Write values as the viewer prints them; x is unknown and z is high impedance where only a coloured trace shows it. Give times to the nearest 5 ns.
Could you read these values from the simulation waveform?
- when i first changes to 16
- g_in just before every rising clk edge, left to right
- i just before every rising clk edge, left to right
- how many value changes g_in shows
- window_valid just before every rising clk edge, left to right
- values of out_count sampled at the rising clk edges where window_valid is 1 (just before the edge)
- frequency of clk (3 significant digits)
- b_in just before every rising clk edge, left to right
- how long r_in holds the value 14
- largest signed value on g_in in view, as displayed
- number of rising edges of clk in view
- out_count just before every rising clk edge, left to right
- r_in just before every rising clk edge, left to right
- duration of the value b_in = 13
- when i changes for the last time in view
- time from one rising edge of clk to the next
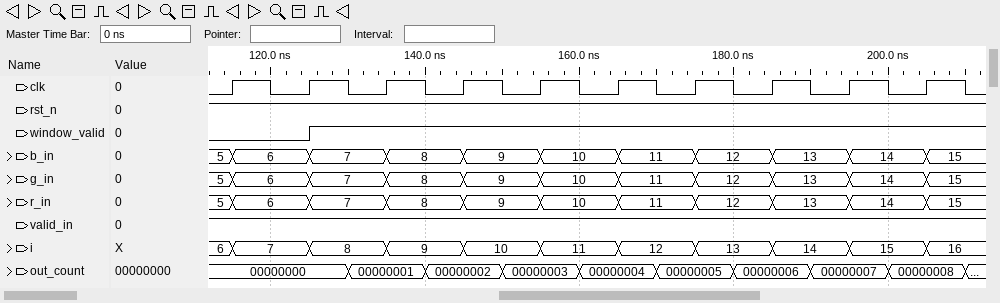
205 ns
5, 6, 7, 8, 9, 10, 11, 12, 13, 14
6, 7, 8, 9, 10, 11, 12, 13, 14, 15
10
0 0 1 1 1 1 1 1 1 1
00000001, 00000002, 00000003, 00000004, 00000005, 00000006, 00000007, 00000008
100 MHz
5, 6, 7, 8, 9, 10, 11, 12, 13, 14
10 ns
15
10
00000000, 00000000, 00000001, 00000002, 00000003, 00000004, 00000005, 00000006, 00000007, 00000008
5, 6, 7, 8, 9, 10, 11, 12, 13, 14
10 ns
205 ns
10 ns
